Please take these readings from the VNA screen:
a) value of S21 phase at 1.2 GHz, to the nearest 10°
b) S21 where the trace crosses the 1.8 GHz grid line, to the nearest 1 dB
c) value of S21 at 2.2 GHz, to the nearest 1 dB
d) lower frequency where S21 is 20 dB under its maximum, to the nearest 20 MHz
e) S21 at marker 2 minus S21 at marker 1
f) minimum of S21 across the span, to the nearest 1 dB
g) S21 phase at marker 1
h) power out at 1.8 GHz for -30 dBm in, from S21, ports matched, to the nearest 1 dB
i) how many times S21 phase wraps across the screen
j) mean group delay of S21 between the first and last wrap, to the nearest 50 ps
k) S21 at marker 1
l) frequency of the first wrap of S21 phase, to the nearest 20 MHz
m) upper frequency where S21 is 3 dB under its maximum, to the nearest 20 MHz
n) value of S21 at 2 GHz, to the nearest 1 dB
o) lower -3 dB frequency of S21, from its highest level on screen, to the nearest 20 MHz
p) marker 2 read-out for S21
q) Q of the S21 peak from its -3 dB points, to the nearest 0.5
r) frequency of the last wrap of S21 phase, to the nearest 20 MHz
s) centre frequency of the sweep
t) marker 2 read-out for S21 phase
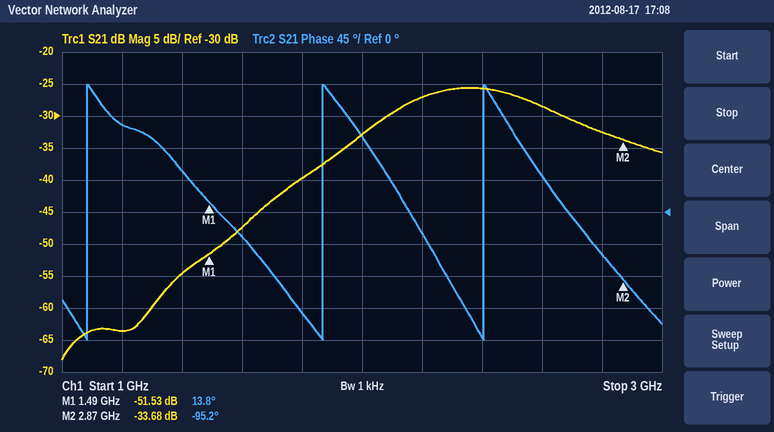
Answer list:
120°
-40 dB
-27 dB
1.64 GHz
17.85 dB
-68 dB
13.8°
-70 dBm
3
1.50 ns
-51.53 dB
1.08 GHz
2.60 GHz
-33 dB
2.14 GHz
-33.68 dB
5.0
2.40 GHz
2 GHz
-95.2°
